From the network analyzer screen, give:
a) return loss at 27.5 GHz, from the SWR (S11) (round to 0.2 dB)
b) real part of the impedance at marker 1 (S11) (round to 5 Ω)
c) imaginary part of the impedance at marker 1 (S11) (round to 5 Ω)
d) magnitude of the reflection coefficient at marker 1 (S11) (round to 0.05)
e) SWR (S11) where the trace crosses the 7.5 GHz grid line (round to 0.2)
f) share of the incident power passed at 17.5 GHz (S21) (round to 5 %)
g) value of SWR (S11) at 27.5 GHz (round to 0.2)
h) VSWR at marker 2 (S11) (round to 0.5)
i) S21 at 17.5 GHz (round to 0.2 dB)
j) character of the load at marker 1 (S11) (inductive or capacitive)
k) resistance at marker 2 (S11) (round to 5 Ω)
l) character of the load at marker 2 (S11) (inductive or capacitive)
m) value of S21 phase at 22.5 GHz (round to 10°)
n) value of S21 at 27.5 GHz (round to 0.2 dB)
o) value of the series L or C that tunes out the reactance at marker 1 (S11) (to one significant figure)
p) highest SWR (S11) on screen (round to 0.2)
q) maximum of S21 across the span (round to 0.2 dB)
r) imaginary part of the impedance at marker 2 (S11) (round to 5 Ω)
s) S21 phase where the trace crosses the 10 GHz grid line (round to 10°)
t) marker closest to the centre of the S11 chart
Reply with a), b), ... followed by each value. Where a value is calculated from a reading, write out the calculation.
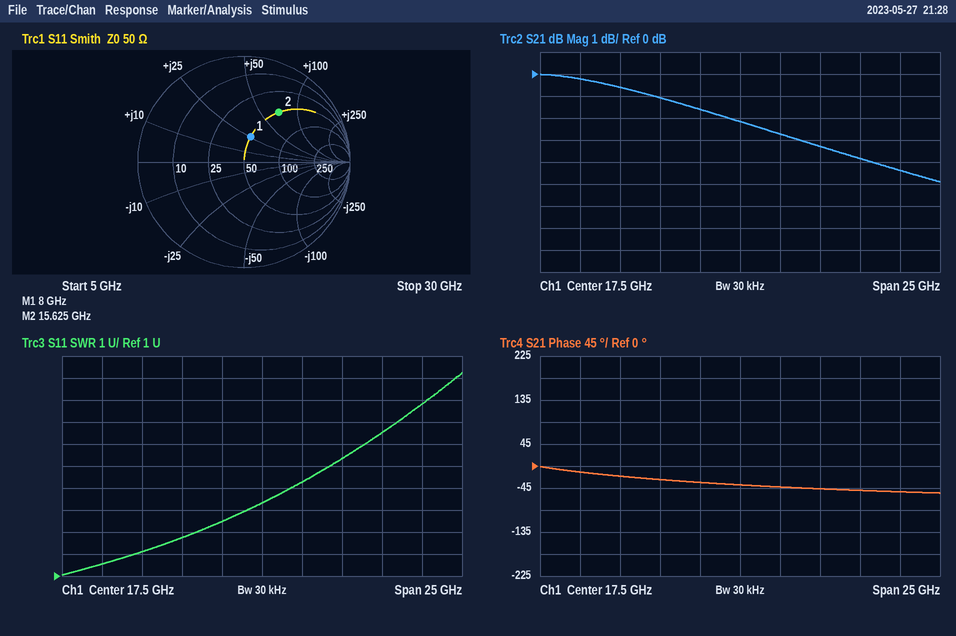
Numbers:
a) −20 log10((8.8 − 1)/(8.8 + 1)) ≈ 2.0 dB
b) 50 Ω
c) +25 Ω
d) 0.25
e) 1.6
f) 10^(-2.2/10) ≈ 60 %
g) 8.8
h) 3.5
i) -2.2 dB
j) inductive
k) 50 Ω
l) inductive
m) -50°
n) -4.4 dB
o) C = 1/(2π × 8 GHz × 25 Ω) ≈ 796 fF, so 800 fF to one significant figure
p) 10.2
q) 0.0 dB
r) +70 Ω
s) -20°
t) marker 1
